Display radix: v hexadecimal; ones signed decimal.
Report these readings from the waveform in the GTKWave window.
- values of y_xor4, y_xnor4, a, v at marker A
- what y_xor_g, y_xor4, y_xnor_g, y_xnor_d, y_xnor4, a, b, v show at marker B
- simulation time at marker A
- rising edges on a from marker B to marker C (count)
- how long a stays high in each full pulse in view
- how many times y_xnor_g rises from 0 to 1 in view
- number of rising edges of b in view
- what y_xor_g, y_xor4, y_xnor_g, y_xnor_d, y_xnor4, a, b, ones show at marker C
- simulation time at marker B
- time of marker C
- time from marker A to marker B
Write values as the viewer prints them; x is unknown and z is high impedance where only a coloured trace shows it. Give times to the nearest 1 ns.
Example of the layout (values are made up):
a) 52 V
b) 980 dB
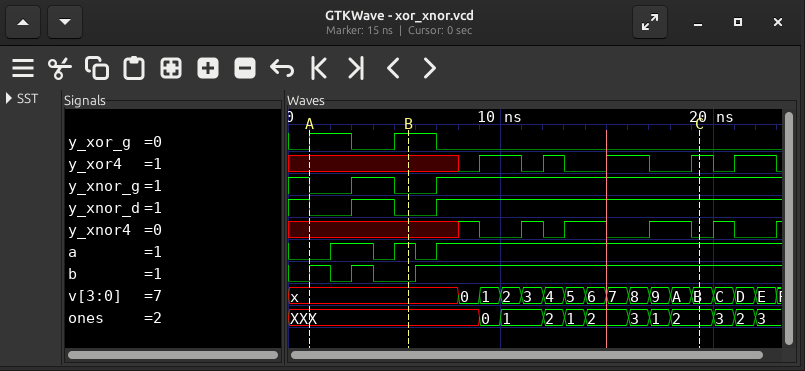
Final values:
a) y_xor4=x, y_xnor4=x, a=0, v=x
b) y_xor_g=1, y_xor4=x, y_xnor_g=0, y_xnor_d=0, y_xnor4=x, a=1, b=0, v=x
c) 1 ns
d) 1
e) 2 ns, 1 ns
f) 2
g) 3
h) y_xor_g=0, y_xor4=1, y_xnor_g=1, y_xnor_d=1, y_xnor4=0, a=1, b=1, ones=2
i) 6 ns
j) 19 ns
k) 5 ns
